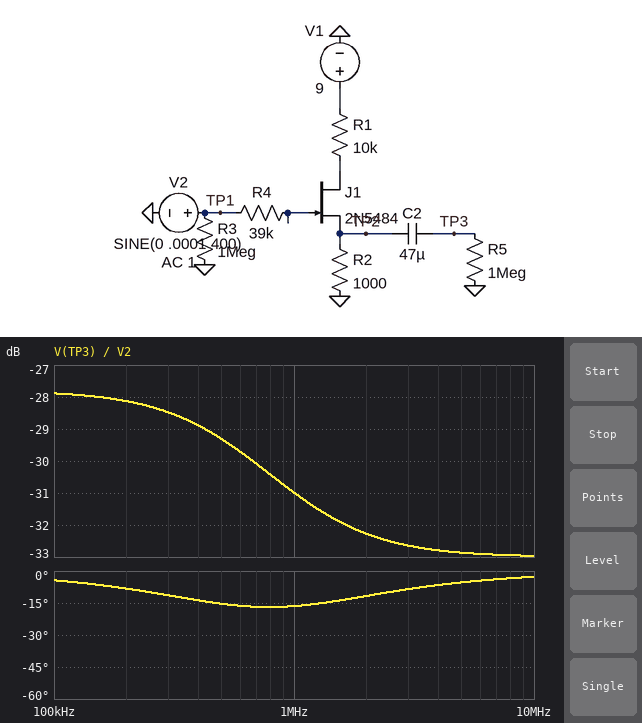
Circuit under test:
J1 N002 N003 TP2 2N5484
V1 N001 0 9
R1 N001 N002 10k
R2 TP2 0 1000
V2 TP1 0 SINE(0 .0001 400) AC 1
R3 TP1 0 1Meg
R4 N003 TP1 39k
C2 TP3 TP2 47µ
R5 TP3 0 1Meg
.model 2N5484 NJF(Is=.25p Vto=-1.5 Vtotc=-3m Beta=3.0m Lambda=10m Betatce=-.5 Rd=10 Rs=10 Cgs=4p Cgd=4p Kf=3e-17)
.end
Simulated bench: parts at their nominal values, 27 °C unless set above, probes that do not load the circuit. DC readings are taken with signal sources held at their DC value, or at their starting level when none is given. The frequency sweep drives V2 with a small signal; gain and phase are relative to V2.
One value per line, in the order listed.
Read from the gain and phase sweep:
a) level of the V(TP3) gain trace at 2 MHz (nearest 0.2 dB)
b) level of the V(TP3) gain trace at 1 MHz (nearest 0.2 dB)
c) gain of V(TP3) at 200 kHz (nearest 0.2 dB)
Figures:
-32.2 dB
-31.0 dB
-28.2 dB
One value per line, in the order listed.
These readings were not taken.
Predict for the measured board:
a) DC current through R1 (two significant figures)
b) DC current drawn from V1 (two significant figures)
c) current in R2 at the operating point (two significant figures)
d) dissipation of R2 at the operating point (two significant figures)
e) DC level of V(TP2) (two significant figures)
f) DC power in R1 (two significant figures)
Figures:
800 µA
800 µA
800 µA
630 µW
800 mV
6.3 mW
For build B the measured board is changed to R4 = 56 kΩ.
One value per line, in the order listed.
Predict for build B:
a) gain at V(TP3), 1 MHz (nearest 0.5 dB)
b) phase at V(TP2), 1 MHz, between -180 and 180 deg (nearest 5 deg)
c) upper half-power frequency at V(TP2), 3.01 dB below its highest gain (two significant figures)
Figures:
-33.5 dB
-25 deg
490 kHz
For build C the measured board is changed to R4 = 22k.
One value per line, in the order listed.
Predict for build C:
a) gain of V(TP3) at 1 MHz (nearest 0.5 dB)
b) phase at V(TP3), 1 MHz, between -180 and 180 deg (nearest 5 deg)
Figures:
-28.0 dB
0 deg
